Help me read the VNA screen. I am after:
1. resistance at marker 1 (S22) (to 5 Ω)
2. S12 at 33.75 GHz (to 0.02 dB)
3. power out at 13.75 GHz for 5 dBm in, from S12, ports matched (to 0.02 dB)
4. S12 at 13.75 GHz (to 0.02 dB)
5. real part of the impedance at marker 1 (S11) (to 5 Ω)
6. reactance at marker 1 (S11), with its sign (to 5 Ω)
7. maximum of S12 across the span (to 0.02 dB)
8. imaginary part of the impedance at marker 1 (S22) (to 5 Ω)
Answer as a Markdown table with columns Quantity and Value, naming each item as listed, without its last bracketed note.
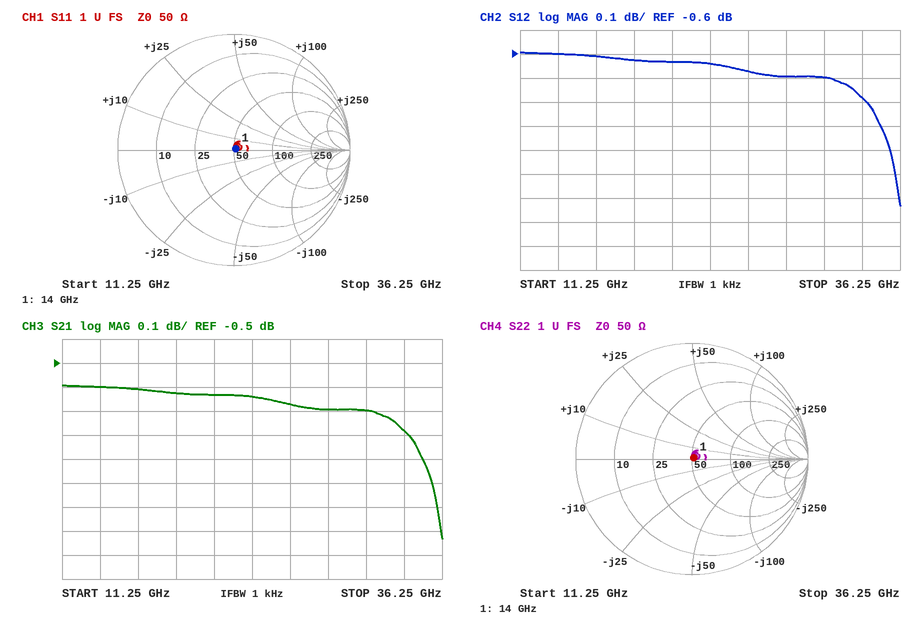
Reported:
| Quantity | Value |
|---|---|
| resistance at marker 1 (S22) | 50 Ω |
| S12 at 33.75 GHz | -0.78 dB |
| power out at 13.75 GHz for 5 dBm in, from S12, ports matched | 4.40 dBm |
| S12 at 13.75 GHz | -0.60 dB |
| real part of the impedance at marker 1 (S11) | 50 Ω |
| reactance at marker 1 (S11), with its sign | 0 Ω |
| maximum of S12 across the span | -0.60 dB |
| imaginary part of the impedance at marker 1 (S22) | 0 Ω |
